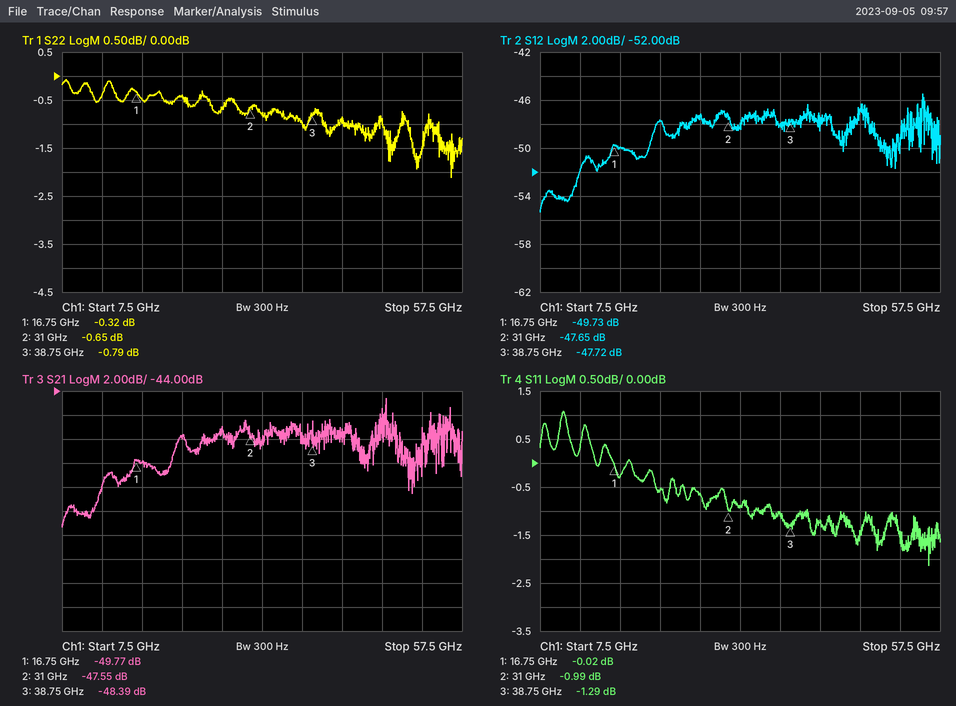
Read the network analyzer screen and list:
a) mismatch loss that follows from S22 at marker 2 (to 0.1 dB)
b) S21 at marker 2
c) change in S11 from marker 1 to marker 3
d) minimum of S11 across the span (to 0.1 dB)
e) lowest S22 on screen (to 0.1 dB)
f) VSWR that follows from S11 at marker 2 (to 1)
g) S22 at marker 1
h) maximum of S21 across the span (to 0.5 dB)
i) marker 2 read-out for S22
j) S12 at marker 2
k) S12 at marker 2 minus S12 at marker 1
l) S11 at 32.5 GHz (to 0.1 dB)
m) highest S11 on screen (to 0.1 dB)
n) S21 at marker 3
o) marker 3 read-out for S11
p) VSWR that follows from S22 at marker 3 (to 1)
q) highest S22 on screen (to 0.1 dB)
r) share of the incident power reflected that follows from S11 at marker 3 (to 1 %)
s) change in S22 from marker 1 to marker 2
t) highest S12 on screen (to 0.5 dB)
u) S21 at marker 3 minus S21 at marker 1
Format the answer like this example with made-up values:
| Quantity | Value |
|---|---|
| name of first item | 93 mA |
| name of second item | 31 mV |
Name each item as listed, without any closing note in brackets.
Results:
| Quantity | Value |
|---|---|
| mismatch loss that follows from S22 at marker 2 | 8.6 dB |
| S21 at marker 2 | -47.55 dB |
| change in S11 from marker 1 to marker 3 | -1.27 dB |
| minimum of S11 across the span | -2.1 dB |
| lowest S22 on screen | -2.1 dB |
| VSWR that follows from S11 at marker 2 | 18 |
| S22 at marker 1 | -0.32 dB |
| maximum of S21 across the span | -44.5 dB |
| marker 2 read-out for S22 | -0.65 dB |
| S12 at marker 2 | -47.65 dB |
| S12 at marker 2 minus S12 at marker 1 | 2.08 dB |
| S11 at 32.5 GHz | -0.9 dB |
| highest S11 on screen | 1.1 dB |
| S21 at marker 3 | -48.39 dB |
| marker 3 read-out for S11 | -1.29 dB |
| VSWR that follows from S22 at marker 3 | 22 |
| highest S22 on screen | -0.1 dB |
| share of the incident power reflected that follows from S11 at marker 3 | 74 % |
| change in S22 from marker 1 to marker 2 | -0.33 dB |
| highest S12 on screen | -45.5 dB |
| S21 at marker 3 minus S21 at marker 1 | 1.38 dB |
